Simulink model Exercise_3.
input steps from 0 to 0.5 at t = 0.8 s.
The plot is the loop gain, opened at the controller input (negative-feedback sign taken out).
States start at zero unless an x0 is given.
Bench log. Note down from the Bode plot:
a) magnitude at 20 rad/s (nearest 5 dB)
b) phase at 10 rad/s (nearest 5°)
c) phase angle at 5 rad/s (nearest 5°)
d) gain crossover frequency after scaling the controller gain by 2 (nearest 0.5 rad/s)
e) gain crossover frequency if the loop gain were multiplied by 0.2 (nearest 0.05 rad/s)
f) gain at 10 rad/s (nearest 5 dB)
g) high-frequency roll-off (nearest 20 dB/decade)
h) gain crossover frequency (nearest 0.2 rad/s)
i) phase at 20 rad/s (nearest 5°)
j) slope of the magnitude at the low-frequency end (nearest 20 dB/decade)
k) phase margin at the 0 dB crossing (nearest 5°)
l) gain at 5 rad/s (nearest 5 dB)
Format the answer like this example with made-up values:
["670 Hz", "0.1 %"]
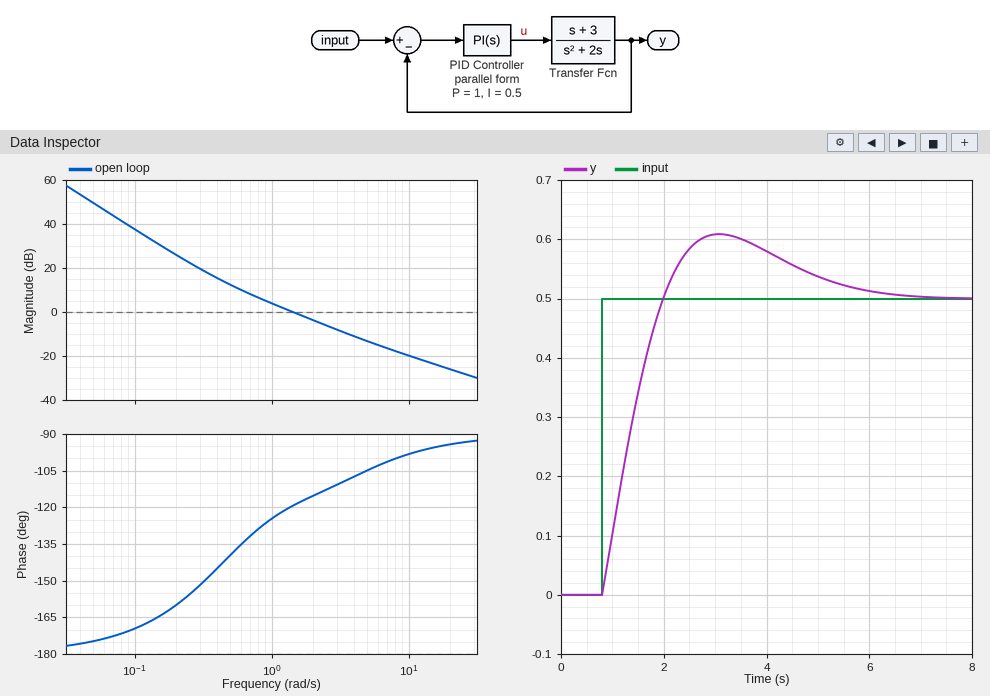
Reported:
["-25 dB", "-100°", "-105°", "2.5 rad/s", "0.45 rad/s", "-20 dB", "-20 dB/decade", "1.4 rad/s", "-95°", "-40 dB/decade", "60°", "-15 dB"]
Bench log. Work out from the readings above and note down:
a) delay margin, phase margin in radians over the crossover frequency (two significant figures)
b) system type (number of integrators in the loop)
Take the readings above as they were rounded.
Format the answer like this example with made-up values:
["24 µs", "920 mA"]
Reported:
["0.75 s", "2"]
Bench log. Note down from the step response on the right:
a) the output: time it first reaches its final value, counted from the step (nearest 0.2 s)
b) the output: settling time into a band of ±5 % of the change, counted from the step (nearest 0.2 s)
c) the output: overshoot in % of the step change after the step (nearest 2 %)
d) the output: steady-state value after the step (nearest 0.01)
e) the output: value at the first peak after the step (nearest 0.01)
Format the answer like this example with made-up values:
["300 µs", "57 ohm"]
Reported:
["1.2 s", "4.6 s", "22 %", "0.50", "0.61"]
